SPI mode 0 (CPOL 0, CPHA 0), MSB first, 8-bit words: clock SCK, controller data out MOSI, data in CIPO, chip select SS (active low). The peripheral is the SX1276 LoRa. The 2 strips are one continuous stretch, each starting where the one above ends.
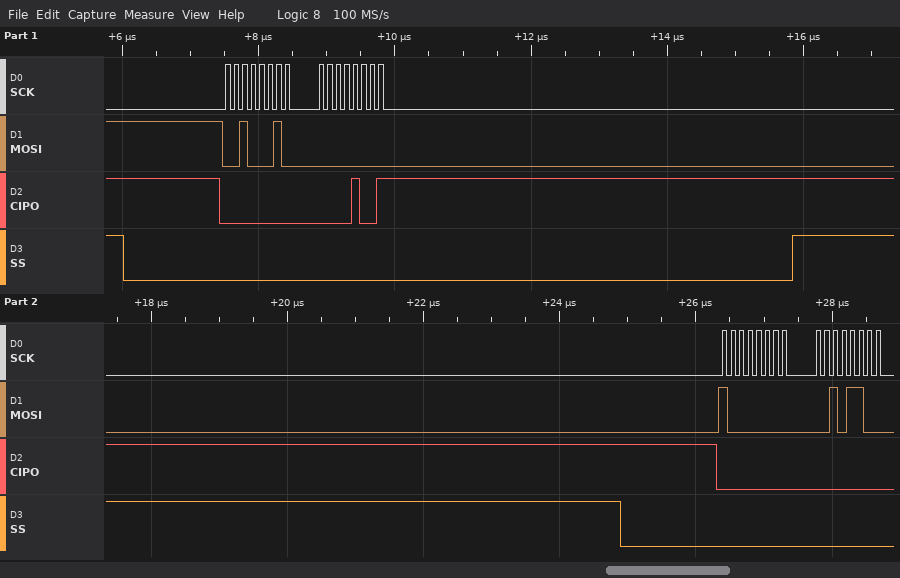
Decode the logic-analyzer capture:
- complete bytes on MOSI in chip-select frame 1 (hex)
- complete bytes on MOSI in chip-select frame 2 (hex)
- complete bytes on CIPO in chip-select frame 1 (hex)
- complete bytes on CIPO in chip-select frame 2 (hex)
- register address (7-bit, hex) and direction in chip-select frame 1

22 00
80 2C
00 09
00 00
0x22 read
